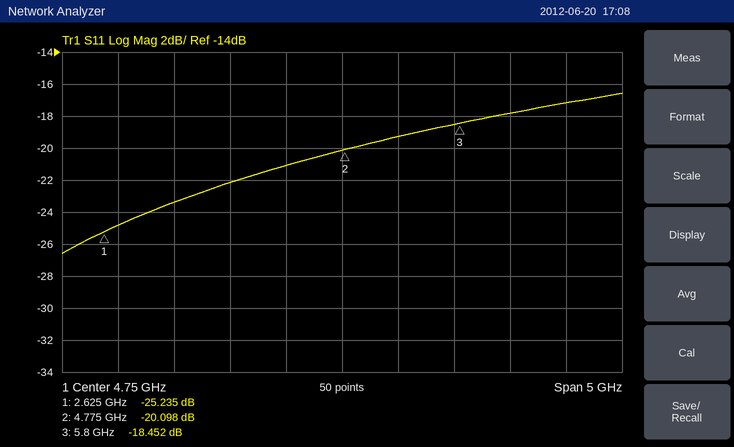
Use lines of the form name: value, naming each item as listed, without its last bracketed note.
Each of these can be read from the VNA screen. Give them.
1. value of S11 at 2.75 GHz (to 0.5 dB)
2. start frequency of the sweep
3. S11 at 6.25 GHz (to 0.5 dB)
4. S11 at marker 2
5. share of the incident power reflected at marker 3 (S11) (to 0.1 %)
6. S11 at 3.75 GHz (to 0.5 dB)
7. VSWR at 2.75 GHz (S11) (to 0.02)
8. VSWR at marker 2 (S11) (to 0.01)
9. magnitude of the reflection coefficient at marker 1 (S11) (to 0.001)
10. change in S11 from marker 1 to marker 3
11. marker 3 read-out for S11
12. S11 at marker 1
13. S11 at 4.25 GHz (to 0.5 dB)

value of S11 at 2.75 GHz: -25.0 dB
start frequency of the sweep: 2.25 GHz
S11 at 6.25 GHz: -18.0 dB
S11 at marker 2: -20.098 dB
share of the incident power reflected at marker 3 (S11): 1.4 %
S11 at 3.75 GHz: -22.0 dB
VSWR at 2.75 GHz (S11): 1.12
VSWR at marker 2 (S11): 1.22
magnitude of the reflection coefficient at marker 1 (S11): 0.055
change in S11 from marker 1 to marker 3: 6.783 dB
marker 3 read-out for S11: -18.452 dB
S11 at marker 1: -25.235 dB
S11 at 4.25 GHz: -21.0 dB
